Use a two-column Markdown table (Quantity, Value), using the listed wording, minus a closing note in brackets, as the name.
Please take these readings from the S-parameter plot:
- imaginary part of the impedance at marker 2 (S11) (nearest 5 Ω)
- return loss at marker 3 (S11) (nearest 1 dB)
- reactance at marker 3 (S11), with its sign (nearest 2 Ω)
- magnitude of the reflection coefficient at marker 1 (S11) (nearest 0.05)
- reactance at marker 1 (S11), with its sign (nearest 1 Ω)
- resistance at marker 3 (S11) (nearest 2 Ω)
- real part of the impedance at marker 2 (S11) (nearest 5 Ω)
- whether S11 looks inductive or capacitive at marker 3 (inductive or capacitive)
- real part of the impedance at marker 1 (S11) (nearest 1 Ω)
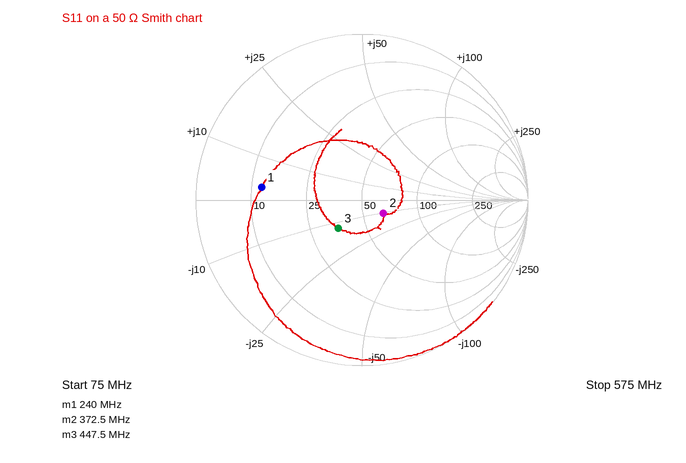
| Quantity | Value |
|---|---|
| imaginary part of the impedance at marker 2 (S11) | -10 Ω |
| return loss at marker 3 (S11) | 13 dB |
| reactance at marker 3 (S11), with its sign | -12 Ω |
| magnitude of the reflection coefficient at marker 1 (S11) | 0.60 |
| reactance at marker 1 (S11), with its sign | +3 Ω |
| resistance at marker 3 (S11) | 36 Ω |
| real part of the impedance at marker 2 (S11) | 65 Ω |
| whether S11 looks inductive or capacitive at marker 3 | capacitive |
| real part of the impedance at marker 1 (S11) | 12 Ω |
